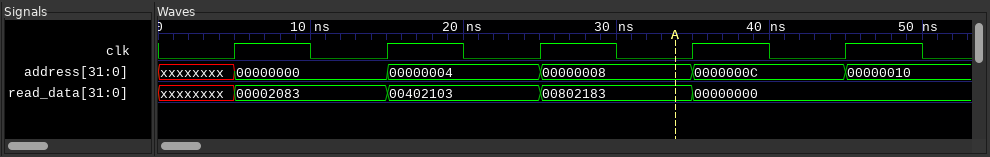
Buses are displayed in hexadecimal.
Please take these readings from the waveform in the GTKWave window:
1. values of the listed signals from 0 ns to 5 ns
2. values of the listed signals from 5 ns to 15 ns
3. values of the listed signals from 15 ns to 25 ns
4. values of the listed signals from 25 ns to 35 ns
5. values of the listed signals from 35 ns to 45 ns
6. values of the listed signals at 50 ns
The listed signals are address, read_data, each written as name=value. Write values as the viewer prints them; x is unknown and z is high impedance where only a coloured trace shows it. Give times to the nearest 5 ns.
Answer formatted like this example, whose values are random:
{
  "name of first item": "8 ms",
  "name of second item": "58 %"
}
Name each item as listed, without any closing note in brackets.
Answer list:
{
  "values of the listed signals from 0 ns to 5 ns": "address=xxxxxxxx, read_data=xxxxxxxx",
  "values of the listed signals from 5 ns to 15 ns": "address=00000000, read_data=00002083",
  "values of the listed signals from 15 ns to 25 ns": "address=00000004, read_data=00402103",
  "values of the listed signals from 25 ns to 35 ns": "address=00000008, read_data=00802183",
  "values of the listed signals from 35 ns to 45 ns": "address=0000000C, read_data=00000000",
  "values of the listed signals at 50 ns": "address=00000010, read_data=00000000"
}
